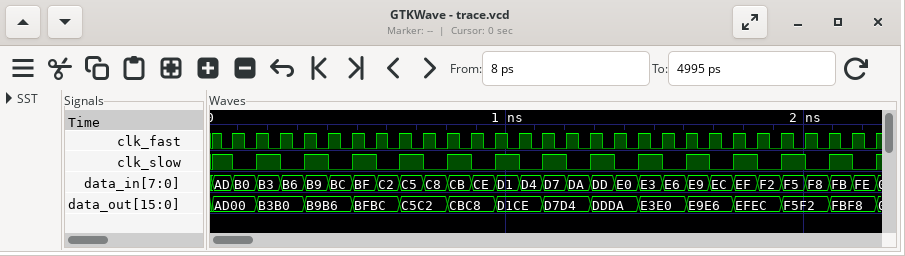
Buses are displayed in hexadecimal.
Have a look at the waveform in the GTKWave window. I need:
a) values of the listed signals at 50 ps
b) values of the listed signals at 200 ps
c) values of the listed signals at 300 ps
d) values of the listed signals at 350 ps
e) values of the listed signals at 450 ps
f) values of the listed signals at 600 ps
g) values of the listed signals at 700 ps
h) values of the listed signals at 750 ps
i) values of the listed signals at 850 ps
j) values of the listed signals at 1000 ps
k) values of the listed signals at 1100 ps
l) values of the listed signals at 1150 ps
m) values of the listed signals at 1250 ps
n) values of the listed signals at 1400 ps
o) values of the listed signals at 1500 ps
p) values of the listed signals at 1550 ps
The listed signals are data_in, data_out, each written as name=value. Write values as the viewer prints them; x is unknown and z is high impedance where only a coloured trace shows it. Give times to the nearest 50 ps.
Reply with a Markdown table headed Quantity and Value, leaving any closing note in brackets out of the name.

| Quantity | Value |
|---|---|
| values of the listed signals at 50 ps | data_in=AD, data_out=AD00 |
| values of the listed signals at 200 ps | data_in=B3, data_out=B3B0 |
| values of the listed signals at 300 ps | data_in=B6, data_out=B3B0 |
| values of the listed signals at 350 ps | data_in=B9, data_out=B9B6 |
| values of the listed signals at 450 ps | data_in=BC, data_out=B9B6 |
| values of the listed signals at 600 ps | data_in=C2, data_out=BFBC |
| values of the listed signals at 700 ps | data_in=C5, data_out=C5C2 |
| values of the listed signals at 750 ps | data_in=C8, data_out=C5C2 |
| values of the listed signals at 850 ps | data_in=CB, data_out=CBC8 |
| values of the listed signals at 1000 ps | data_in=D1, data_out=D1CE |
| values of the listed signals at 1100 ps | data_in=D4, data_out=D1CE |
| values of the listed signals at 1150 ps | data_in=D7, data_out=D7D4 |
| values of the listed signals at 1250 ps | data_in=DA, data_out=D7D4 |
| values of the listed signals at 1400 ps | data_in=E0, data_out=DDDA |
| values of the listed signals at 1500 ps | data_in=E3, data_out=E3E0 |
| values of the listed signals at 1550 ps | data_in=E6, data_out=E3E0 |
